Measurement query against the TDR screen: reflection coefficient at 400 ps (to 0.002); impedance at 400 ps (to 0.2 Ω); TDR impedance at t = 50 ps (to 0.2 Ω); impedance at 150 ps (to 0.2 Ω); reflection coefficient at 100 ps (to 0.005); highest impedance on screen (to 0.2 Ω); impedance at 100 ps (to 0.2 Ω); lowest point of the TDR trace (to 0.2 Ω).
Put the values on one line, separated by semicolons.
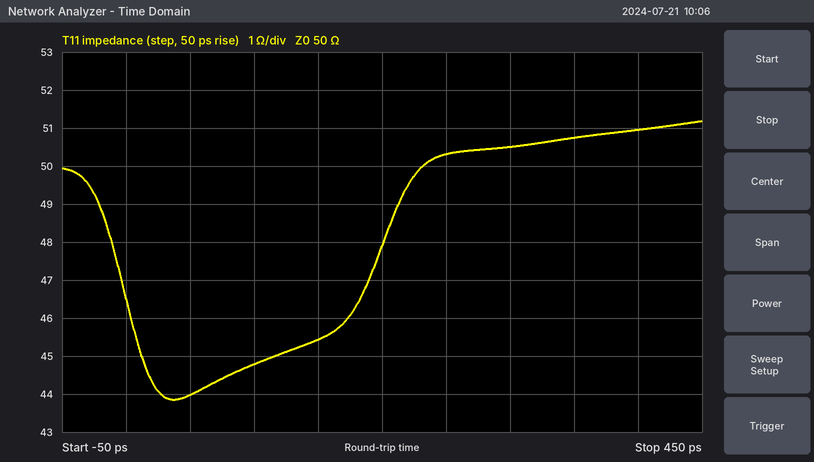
+0.010; 51.0 Ω; 44.0 Ω; 45.4 Ω; -0.055; 51.2 Ω; 44.8 Ω; 43.8 Ω
